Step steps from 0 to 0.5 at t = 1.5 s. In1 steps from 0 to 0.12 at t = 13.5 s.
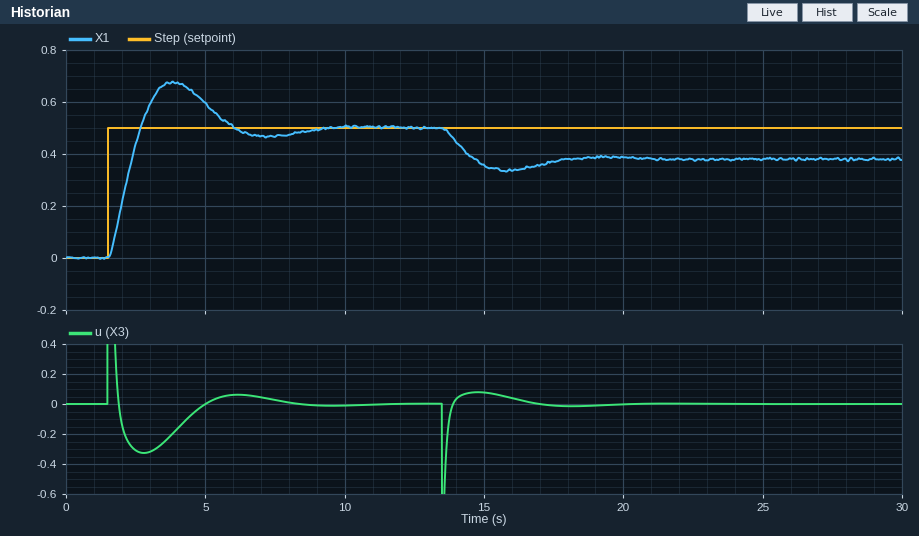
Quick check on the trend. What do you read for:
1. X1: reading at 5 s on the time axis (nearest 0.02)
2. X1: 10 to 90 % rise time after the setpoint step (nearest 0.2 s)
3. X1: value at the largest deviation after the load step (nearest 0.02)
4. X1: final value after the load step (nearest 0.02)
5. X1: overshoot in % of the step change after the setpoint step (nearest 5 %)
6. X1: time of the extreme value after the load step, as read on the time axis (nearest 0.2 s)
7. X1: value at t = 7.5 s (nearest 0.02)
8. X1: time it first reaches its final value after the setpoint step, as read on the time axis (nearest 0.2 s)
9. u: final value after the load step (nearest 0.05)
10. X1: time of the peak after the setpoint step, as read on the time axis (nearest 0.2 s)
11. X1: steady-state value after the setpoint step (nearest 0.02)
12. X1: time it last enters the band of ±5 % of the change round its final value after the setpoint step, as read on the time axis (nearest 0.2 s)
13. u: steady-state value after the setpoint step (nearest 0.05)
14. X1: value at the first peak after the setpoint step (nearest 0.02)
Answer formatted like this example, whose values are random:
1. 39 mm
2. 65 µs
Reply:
1. 0.60
2. 0.8 s
3. 0.34
4. 0.38
5. 35 %
6. 15.8 s
7. 0.46
8. 2.6 s
9. 0.00
10. 3.8 s
11. 0.50
12. 8.0 s
13. 0.00
14. 0.68
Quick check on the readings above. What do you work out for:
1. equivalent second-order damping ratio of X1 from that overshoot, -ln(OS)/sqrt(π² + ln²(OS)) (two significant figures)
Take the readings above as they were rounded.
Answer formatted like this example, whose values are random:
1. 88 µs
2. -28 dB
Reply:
1. 0.32
